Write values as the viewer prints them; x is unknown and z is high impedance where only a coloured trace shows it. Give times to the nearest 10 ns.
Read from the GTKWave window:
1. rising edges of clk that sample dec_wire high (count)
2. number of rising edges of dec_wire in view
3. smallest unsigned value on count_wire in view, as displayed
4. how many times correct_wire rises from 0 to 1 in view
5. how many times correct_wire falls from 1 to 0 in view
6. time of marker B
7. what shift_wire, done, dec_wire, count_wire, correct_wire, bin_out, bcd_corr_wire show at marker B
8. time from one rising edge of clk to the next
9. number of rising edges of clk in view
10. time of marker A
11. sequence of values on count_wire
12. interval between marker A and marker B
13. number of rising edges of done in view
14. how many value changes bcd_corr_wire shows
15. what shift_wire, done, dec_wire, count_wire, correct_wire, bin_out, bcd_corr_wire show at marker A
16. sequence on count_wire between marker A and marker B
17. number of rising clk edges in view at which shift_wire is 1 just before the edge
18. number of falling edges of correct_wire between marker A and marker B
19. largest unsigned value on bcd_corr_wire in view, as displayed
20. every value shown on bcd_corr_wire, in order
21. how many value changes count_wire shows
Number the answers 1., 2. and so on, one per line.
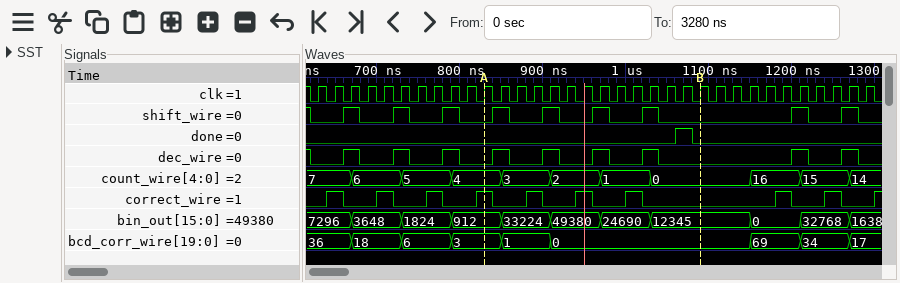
1. 9
2. 9
3. 0
4. 10
5. 9
6. 1090 ns
7. shift_wire=0, done=0, dec_wire=0, count_wire=0, correct_wire=0, bin_out=12345, bcd_corr_wire=0
8. 20 ns
9. 34
10. 830 ns
11. 7, 6, 5, 4, 3, 2, 1, 0, 16, 15, 14
12. 260 ns
13. 1
14. 8
15. shift_wire=0, done=0, dec_wire=0, count_wire=4, correct_wire=1, bin_out=912, bcd_corr_wire=3
16. 4, 3, 2, 1, 0
17. 9
18. 4
19. 69
20. 36, 18, 6, 3, 1, 0, 69, 34, 17
21. 10
